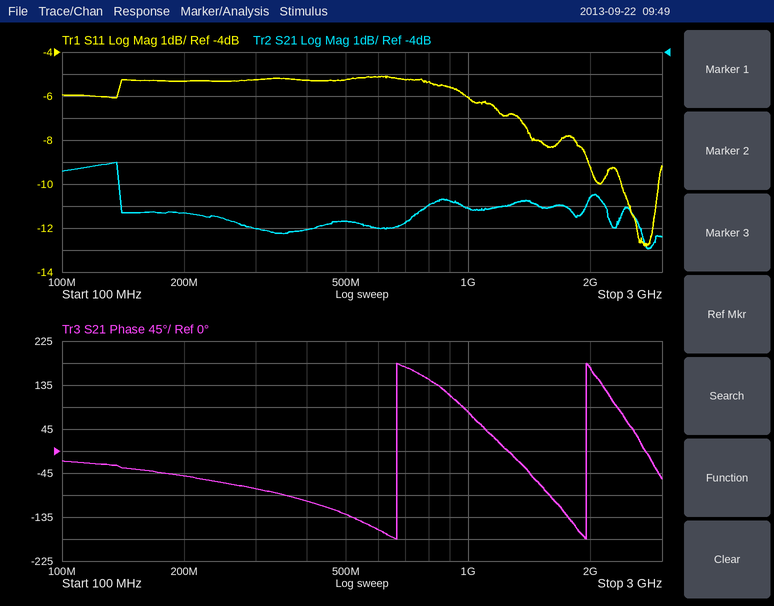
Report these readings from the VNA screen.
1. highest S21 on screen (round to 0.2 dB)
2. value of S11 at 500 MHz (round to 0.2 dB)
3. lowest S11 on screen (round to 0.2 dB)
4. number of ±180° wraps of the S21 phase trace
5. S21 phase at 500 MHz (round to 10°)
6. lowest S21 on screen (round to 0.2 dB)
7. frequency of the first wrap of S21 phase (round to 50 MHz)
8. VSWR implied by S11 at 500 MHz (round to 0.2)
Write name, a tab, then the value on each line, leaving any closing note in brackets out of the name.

highest S21 on screen	-9.0 dB
value of S11 at 500 MHz	-5.2 dB
lowest S11 on screen	-12.8 dB
number of ±180° wraps of the S21 phase trace	2
S21 phase at 500 MHz	-130°
lowest S21 on screen	-13.0 dB
frequency of the first wrap of S21 phase	650 MHz
VSWR implied by S11 at 500 MHz	3.4
